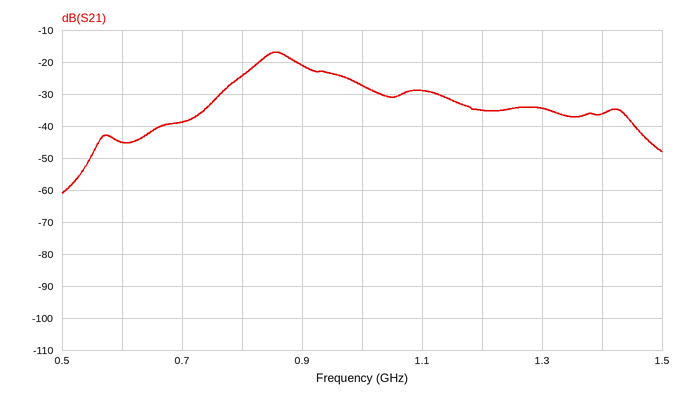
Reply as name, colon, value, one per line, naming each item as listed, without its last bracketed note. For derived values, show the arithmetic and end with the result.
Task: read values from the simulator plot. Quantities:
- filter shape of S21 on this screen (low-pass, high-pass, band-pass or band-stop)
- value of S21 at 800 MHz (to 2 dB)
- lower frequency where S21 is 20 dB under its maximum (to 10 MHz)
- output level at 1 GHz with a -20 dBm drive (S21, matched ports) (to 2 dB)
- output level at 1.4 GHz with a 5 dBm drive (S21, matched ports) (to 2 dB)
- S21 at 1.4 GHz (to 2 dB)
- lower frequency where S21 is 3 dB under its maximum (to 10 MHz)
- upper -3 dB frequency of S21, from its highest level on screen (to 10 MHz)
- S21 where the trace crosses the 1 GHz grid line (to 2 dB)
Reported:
filter shape of S21 on this screen: band-pass
value of S21 at 800 MHz: -24 dB
lower frequency where S21 is 20 dB under its maximum: 720 MHz
output level at 1 GHz with a -20 dBm drive (S21, matched ports): -20 dBm + (-28 dB) = -48 dBm
output level at 1.4 GHz with a 5 dBm drive (S21, matched ports): 5 dBm + (-36 dB) = -32 dBm
S21 at 1.4 GHz: -36 dB
lower frequency where S21 is 3 dB under its maximum: 830 MHz
upper -3 dB frequency of S21, from its highest level on screen: 890 MHz
S21 where the trace crosses the 1 GHz grid line: -28 dB
